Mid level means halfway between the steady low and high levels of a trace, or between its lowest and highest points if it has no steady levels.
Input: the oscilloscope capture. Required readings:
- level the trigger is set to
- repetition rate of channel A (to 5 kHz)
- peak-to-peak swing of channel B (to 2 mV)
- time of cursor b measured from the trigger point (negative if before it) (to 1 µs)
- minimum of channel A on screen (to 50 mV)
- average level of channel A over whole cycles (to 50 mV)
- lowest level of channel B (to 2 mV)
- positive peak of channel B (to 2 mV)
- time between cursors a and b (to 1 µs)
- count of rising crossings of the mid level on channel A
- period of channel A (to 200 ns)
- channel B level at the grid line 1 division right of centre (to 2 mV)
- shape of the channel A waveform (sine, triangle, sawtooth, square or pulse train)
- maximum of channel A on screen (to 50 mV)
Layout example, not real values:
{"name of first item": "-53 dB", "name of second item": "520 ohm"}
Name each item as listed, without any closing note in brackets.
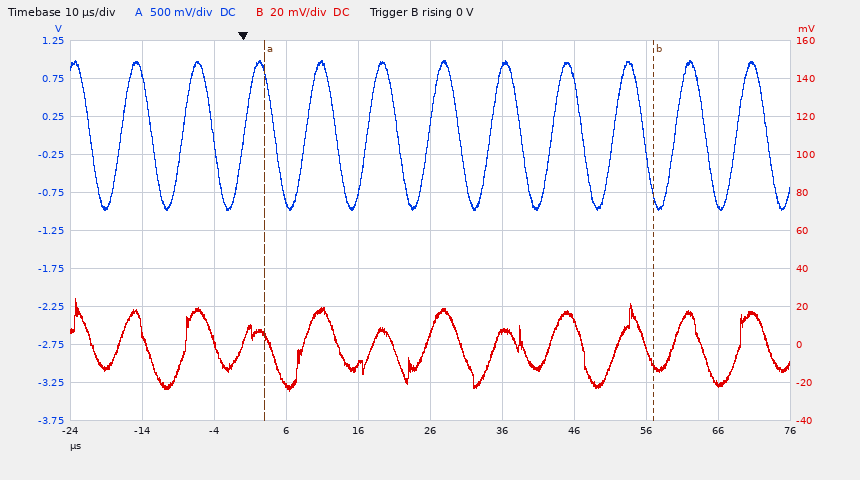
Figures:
{"level the trigger is set to": "0 V", "repetition rate of channel A": "115 kHz", "peak-to-peak swing of channel B": "48 mV", "time of cursor b measured from the trigger point (negative if before it)": "+57 µs", "minimum of channel A on screen": "-1.00 V", "average level of channel A over whole cycles": "0 mV", "lowest level of channel B": "-24 mV", "positive peak of channel B": "24 mV", "time between cursors a and b": "54 µs", "count of rising crossings of the mid level on channel A": "11", "period of channel A": "8.6 µs", "channel B level at the grid line 1 division right of centre": "6 mV", "shape of the channel A waveform": "sine", "maximum of channel A on screen": "1.00 V"}
